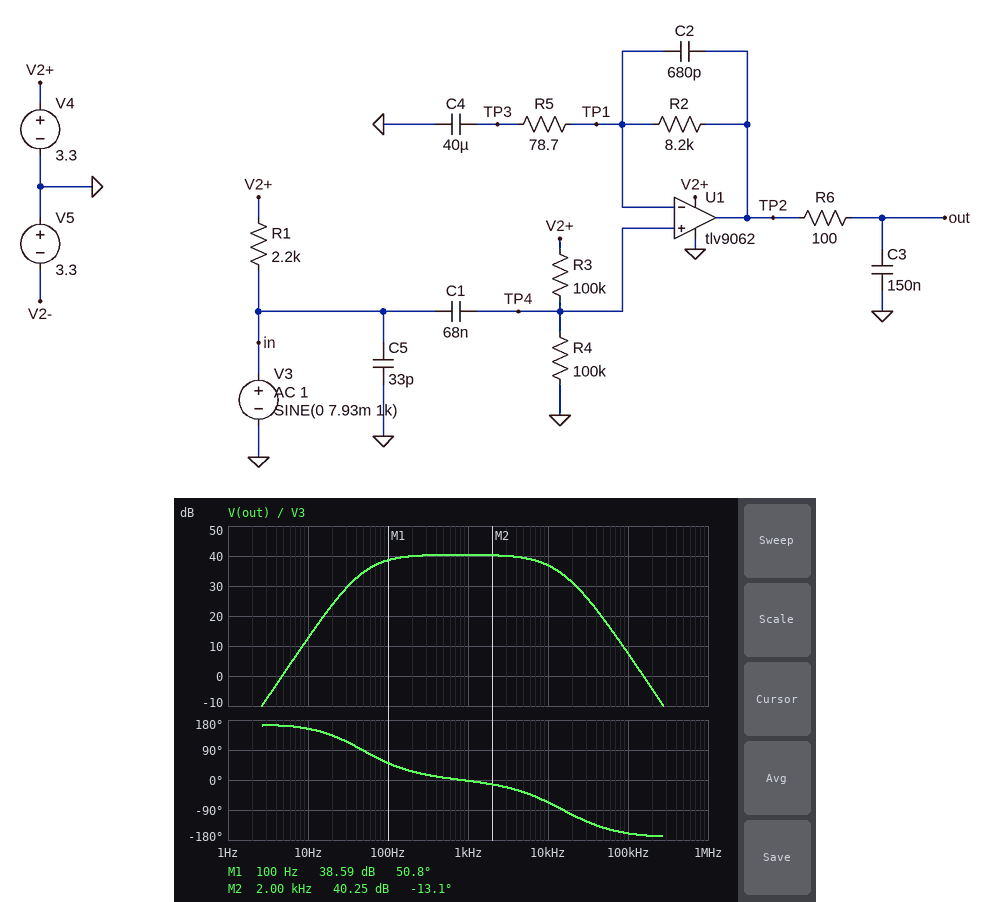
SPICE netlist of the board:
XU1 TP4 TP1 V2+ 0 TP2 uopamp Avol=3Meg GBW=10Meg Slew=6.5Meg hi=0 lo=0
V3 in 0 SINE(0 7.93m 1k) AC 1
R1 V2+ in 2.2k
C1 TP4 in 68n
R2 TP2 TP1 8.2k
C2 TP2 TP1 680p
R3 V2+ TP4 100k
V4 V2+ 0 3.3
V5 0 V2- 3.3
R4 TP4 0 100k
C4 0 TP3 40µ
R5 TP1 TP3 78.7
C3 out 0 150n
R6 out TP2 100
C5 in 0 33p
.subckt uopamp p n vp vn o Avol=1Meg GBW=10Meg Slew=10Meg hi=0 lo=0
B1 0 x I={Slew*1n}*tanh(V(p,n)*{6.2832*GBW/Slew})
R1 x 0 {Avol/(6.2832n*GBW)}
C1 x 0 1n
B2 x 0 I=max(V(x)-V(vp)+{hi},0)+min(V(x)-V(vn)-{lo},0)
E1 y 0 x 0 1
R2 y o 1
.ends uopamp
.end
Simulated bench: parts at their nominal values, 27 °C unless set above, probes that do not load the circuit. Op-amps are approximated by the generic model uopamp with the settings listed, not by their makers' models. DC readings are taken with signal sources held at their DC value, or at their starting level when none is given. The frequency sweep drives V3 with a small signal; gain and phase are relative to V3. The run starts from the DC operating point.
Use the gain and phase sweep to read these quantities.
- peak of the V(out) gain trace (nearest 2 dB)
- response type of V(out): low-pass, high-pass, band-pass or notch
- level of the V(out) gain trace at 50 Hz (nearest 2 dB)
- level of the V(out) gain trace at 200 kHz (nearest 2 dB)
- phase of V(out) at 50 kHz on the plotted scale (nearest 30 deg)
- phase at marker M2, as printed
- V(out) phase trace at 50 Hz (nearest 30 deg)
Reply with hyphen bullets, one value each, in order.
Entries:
- 40 dB
- band-pass
- 34 dB
- -4 dB
- -150 deg
- -13.1 deg
- 90 deg
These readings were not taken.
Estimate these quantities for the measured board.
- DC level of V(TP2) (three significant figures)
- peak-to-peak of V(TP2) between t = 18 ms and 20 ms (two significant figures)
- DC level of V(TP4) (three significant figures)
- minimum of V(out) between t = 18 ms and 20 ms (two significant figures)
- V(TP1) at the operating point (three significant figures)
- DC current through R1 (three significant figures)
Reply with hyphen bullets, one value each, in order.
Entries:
- 1.65 V
- 1.7 V
- 1.65 V
- 820 mV
- 1.65 V
- 1.50 mA
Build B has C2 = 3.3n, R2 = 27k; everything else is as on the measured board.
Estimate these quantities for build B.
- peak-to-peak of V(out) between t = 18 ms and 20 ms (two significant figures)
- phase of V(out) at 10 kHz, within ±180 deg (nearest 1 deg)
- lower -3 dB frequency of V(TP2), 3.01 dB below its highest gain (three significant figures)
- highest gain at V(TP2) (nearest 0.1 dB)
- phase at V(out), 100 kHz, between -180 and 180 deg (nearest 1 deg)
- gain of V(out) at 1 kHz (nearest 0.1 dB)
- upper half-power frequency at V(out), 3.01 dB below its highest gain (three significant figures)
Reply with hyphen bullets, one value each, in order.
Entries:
- 3.3 V
- -122 deg
- 71.0 Hz
- 50.4 dB
- -164 deg
- 49.4 dB
- 1.77 kHz
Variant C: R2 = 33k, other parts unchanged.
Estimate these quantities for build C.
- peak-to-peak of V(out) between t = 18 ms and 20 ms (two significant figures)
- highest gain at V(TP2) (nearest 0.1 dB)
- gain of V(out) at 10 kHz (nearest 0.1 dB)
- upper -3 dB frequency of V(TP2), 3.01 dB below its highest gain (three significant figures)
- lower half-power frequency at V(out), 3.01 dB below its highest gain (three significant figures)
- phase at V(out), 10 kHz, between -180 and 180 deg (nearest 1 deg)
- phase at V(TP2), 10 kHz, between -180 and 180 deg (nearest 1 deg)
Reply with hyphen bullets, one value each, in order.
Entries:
- 3.3 V
- 52.4 dB
- 43.3 dB
- 5.59 kHz
- 74.0 Hz
- -104 deg
- -61 deg
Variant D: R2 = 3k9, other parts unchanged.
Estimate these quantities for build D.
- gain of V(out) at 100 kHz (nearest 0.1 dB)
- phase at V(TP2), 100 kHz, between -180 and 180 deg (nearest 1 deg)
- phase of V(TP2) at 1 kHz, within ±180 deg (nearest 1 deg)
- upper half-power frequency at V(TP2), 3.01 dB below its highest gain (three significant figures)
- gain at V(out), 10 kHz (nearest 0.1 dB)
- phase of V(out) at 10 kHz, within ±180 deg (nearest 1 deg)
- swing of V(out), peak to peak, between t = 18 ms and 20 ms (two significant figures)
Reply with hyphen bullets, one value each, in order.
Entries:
- 7.0 dB
- -64 deg
- 4 deg
- 46.3 kHz
- 31.1 dB
- -55 deg
- 800 mV
